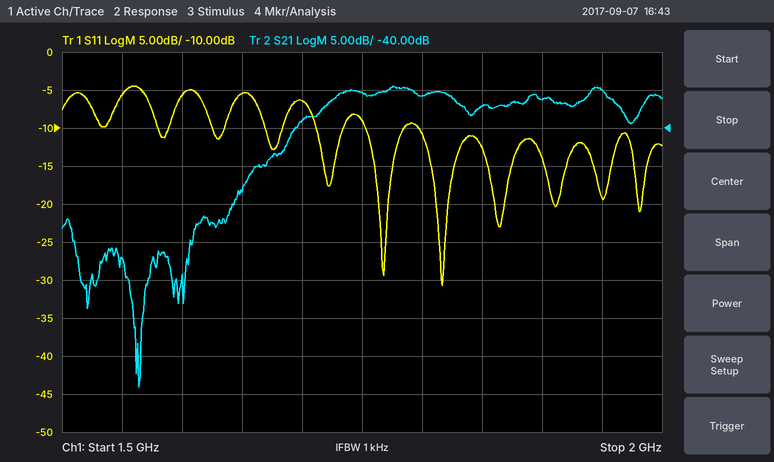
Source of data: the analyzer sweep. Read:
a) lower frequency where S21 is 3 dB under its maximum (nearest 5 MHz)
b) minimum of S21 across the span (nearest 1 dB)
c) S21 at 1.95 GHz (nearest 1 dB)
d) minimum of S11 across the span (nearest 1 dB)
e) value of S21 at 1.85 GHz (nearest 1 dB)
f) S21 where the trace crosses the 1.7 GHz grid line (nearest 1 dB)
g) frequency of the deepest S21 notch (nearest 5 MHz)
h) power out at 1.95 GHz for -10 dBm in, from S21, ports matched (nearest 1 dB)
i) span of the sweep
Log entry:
1.715 GHz
-74 dB
-35 dB
-31 dB
-37 dB
-39 dB
1.565 GHz
-45 dBm
500 MHz
